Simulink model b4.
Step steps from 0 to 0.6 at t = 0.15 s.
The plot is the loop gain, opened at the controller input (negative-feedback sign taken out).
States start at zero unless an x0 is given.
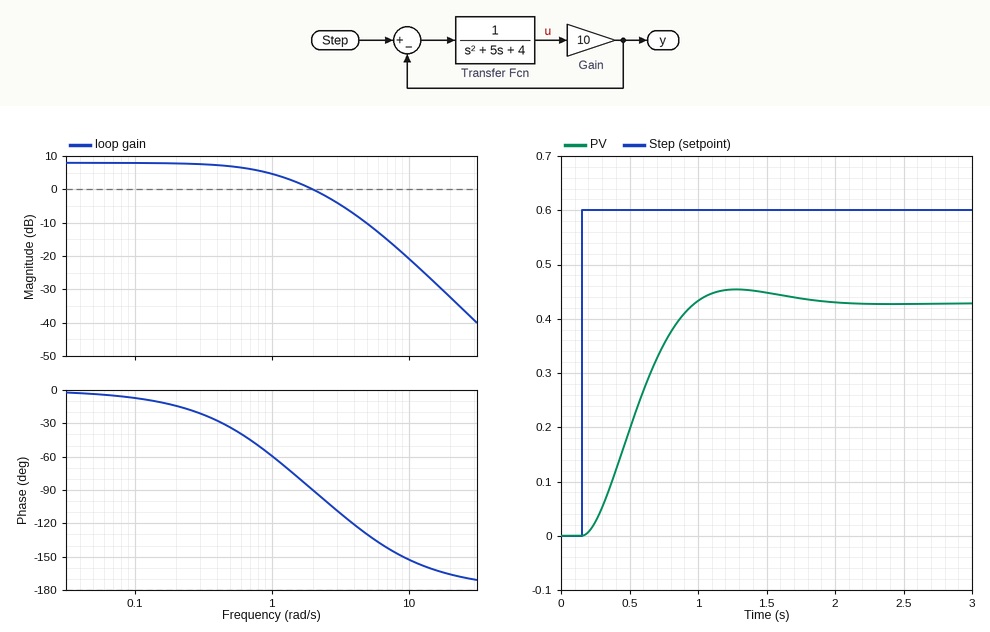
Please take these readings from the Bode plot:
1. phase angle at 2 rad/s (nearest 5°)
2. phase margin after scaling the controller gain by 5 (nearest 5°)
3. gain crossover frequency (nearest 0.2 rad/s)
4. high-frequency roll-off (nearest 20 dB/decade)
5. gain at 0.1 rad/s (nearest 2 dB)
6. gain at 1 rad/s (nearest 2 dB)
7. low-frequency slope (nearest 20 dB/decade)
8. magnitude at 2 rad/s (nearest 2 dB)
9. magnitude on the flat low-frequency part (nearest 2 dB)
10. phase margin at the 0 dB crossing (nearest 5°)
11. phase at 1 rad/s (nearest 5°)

-90°
40°
2.0 rad/s
-40 dB/decade
8 dB
4 dB
0 dB/decade
0 dB
8 dB
90°
-60°
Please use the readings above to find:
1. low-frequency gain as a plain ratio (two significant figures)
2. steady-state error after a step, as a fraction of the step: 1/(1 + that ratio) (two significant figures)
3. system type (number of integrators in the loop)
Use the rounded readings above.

2.5
0.29
0
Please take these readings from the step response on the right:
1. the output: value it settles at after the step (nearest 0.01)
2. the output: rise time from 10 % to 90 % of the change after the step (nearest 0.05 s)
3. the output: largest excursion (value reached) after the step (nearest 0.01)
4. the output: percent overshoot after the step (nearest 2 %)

0.43
0.55 s
0.45
6 %
